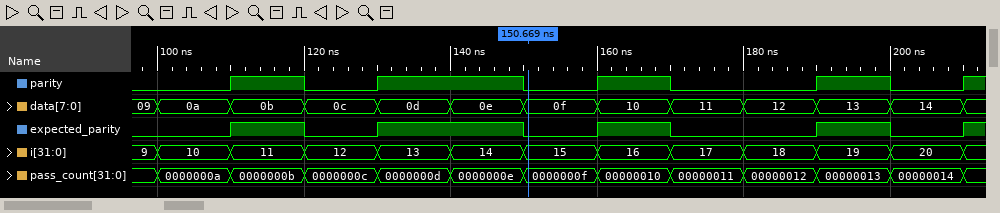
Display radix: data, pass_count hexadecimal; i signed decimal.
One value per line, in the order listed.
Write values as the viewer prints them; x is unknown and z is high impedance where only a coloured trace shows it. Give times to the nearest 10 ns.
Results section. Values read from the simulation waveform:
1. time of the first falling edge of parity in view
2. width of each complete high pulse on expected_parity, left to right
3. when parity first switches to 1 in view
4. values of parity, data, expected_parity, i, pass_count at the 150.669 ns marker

120 ns
10 ns, 20 ns, 10 ns, 10 ns
110 ns
parity=0, data=0f, expected_parity=0, i=15, pass_count=0000000f
